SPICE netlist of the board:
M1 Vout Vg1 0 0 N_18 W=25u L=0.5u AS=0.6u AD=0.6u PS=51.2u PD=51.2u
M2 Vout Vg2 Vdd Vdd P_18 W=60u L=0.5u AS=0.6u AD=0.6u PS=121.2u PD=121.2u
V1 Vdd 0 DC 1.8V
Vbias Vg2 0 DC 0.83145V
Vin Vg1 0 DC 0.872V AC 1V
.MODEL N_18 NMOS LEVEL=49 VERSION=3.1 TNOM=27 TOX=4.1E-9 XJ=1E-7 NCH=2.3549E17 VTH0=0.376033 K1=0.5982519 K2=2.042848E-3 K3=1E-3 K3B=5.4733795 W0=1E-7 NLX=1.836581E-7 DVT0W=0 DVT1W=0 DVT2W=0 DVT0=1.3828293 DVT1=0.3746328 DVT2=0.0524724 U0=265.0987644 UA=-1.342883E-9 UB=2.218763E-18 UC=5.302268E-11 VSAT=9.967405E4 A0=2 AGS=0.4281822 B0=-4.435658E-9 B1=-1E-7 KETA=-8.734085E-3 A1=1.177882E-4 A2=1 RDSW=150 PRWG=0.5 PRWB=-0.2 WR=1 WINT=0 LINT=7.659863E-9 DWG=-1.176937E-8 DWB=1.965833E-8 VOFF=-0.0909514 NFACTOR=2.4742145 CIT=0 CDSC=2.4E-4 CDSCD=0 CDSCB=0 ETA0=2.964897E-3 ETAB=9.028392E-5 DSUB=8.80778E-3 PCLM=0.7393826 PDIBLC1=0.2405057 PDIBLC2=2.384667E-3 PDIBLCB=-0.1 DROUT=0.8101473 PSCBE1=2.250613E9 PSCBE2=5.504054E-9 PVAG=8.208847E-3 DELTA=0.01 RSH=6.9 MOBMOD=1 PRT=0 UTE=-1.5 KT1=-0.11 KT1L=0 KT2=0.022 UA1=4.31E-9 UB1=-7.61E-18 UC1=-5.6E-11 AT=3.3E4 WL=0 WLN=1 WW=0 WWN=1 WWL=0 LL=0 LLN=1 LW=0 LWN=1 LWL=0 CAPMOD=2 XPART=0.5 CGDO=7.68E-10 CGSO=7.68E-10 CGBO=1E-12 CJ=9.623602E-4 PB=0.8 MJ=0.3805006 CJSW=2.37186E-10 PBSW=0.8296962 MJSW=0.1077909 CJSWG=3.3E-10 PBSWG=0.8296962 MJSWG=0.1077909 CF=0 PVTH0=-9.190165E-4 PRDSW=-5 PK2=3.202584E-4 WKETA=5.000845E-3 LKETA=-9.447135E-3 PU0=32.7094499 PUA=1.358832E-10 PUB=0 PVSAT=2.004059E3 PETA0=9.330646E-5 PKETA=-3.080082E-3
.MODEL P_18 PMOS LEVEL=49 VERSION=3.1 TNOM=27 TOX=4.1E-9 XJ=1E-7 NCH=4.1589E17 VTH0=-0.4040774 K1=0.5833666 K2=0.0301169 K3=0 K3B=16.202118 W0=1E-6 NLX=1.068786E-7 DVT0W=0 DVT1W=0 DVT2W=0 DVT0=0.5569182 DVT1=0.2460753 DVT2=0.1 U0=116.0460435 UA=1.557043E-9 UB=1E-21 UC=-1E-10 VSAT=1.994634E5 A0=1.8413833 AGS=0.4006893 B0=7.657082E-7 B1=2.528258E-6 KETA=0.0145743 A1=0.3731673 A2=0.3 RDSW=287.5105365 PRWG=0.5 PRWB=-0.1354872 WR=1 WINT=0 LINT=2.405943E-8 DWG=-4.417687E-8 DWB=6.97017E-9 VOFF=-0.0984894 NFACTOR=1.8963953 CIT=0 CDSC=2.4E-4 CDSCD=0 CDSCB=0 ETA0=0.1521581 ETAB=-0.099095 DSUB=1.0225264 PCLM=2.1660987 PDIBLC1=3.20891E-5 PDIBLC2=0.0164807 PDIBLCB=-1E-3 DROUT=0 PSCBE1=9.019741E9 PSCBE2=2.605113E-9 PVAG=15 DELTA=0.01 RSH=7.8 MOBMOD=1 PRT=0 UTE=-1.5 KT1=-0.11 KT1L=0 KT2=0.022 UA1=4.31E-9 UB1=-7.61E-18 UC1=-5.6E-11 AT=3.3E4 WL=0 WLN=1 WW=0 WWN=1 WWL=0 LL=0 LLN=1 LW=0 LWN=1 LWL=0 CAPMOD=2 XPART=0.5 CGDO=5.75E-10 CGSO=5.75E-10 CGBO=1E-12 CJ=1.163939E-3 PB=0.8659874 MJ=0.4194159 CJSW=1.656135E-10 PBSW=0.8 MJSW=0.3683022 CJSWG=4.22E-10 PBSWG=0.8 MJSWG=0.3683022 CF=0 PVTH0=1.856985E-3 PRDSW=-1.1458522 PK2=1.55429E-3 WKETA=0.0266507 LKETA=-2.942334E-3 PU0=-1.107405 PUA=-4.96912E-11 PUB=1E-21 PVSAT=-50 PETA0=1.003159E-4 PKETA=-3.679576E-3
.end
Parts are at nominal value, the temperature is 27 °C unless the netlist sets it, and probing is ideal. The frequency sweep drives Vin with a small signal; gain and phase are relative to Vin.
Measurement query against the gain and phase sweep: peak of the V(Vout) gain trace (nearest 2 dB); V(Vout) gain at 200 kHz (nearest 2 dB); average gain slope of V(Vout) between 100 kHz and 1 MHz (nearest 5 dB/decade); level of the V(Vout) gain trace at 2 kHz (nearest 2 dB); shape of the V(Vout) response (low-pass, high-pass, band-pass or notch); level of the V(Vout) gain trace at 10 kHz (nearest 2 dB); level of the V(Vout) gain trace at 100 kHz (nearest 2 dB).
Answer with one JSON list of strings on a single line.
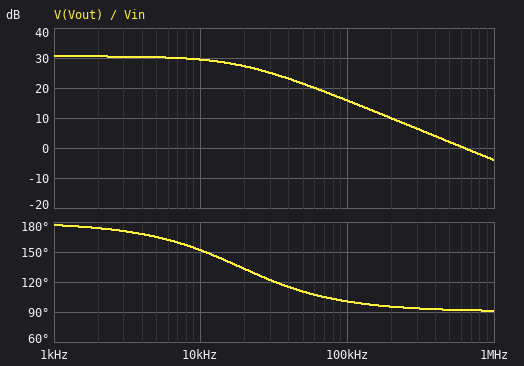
["30 dB", "10 dB", "-20 dB/decade", "30 dB", "low-pass", "30 dB", "16 dB"]
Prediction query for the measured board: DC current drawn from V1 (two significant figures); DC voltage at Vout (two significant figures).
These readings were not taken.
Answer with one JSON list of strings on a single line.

["870 µA", "920 mV"]
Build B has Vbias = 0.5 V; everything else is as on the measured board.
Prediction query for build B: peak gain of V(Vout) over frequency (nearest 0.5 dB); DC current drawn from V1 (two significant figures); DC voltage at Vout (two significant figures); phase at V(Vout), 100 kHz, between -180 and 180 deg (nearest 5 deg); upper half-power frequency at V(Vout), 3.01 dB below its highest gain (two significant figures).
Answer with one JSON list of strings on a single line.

["-1.0 dB", "900 µA", "1.6 V", "170 deg", "670 kHz"]
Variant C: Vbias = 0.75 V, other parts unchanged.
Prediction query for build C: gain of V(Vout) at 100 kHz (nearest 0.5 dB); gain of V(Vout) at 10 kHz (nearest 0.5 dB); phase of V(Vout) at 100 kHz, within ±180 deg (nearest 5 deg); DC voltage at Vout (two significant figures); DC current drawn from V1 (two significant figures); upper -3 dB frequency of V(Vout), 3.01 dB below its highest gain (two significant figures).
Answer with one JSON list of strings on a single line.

["6.5 dB", "7.0 dB", "160 deg", "1.5 V", "900 µA", "270 kHz"]
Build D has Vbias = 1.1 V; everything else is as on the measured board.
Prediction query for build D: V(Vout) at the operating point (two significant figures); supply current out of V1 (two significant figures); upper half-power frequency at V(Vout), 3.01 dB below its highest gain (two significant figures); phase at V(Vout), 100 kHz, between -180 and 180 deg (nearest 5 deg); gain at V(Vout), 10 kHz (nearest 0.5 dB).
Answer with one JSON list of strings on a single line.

["54 mV", "250 µA", "680 kHz", "170 deg", "-16.5 dB"]
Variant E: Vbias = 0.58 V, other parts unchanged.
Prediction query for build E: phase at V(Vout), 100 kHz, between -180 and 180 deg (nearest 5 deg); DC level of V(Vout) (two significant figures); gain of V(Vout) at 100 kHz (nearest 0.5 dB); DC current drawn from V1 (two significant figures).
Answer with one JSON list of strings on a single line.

["170 deg", "1.6 V", "0.5 dB", "900 µA"]
